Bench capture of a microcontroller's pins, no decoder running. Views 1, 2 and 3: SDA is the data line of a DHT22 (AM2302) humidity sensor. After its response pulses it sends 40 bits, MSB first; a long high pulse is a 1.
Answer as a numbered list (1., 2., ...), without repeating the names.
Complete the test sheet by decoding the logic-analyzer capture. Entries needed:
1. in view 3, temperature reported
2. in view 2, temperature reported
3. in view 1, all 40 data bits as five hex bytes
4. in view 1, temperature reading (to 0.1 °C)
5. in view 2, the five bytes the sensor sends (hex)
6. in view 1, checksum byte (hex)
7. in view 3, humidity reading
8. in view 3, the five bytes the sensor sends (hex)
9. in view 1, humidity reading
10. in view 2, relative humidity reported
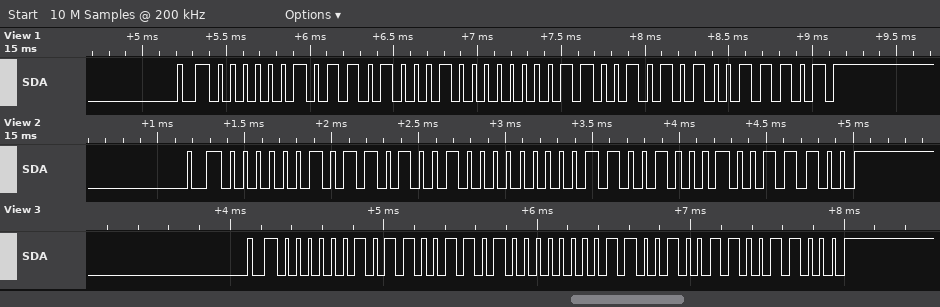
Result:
1. 20.1 °C
2. 20.0 °C
3. 02 D1 00 CA 9D
4. 20.2 °C
5. 02 D2 00 C8 9C
6. 0x9D
7. 71.7 %
8. 02 CD 00 C9 98
9. 72.1 %
10. 72.2 %
